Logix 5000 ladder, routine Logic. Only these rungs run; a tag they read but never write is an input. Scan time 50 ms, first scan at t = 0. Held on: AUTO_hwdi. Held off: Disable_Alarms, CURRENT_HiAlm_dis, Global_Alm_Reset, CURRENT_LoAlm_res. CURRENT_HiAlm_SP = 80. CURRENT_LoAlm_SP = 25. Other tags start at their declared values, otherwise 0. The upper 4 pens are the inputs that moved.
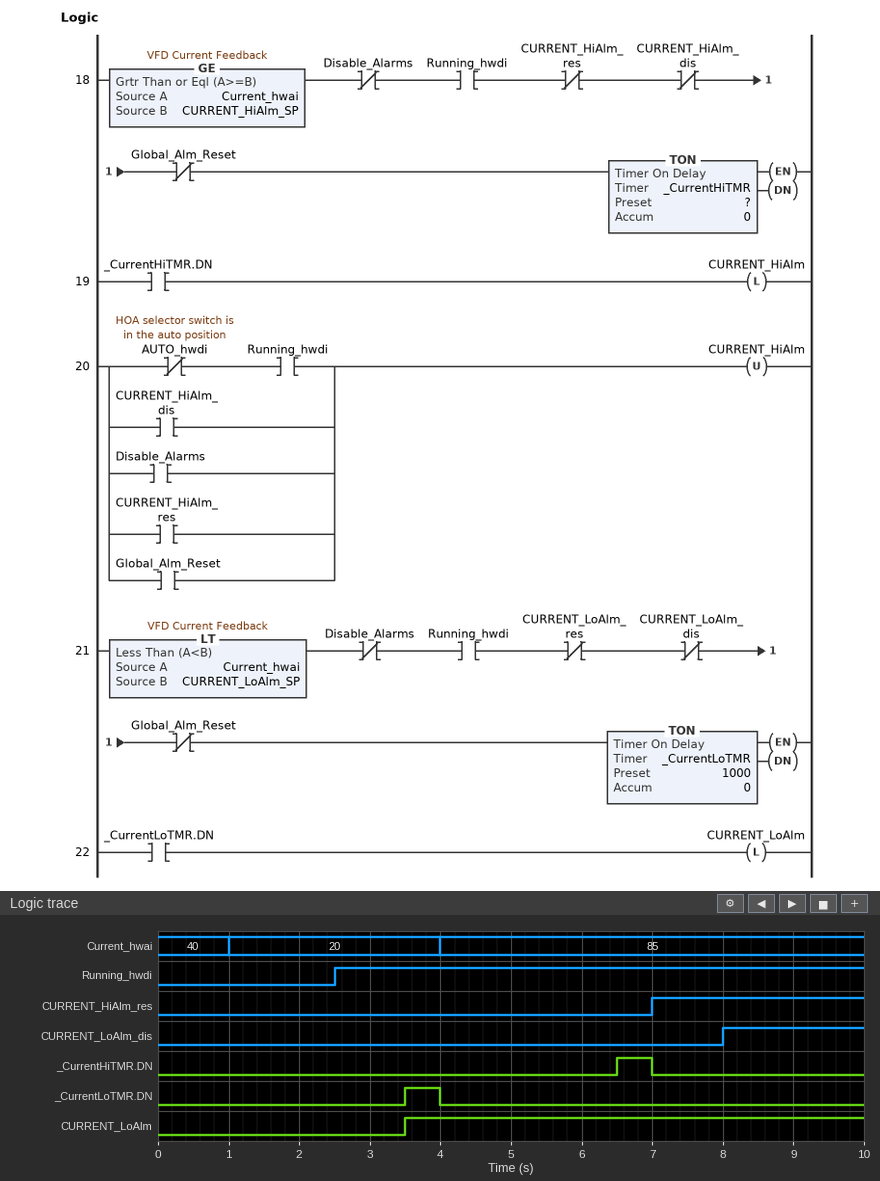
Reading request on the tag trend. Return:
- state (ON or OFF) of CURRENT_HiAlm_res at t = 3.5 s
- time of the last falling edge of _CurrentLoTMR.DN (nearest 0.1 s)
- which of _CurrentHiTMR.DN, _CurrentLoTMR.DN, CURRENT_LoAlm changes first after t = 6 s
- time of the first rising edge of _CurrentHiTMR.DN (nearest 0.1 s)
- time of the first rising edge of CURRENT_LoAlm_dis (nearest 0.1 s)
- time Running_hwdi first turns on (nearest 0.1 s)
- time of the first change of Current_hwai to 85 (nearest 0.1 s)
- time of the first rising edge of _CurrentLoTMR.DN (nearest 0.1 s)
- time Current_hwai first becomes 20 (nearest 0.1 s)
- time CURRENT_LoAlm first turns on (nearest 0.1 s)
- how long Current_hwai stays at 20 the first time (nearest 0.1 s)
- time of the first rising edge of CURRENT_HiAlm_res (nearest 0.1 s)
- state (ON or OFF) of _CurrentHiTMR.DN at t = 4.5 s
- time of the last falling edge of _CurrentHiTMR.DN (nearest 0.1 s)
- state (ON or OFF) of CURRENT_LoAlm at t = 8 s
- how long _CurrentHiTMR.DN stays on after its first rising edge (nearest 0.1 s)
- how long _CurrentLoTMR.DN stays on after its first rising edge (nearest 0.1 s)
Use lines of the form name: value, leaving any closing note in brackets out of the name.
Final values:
state (ON or OFF) of CURRENT_HiAlm_res at t = 3.5 s: OFF
time of the last falling edge of _CurrentLoTMR.DN: 4.0 s
which of _CurrentHiTMR.DN, _CurrentLoTMR.DN, CURRENT_LoAlm changes first after t = 6 s: _CurrentHiTMR.DN
time of the first rising edge of _CurrentHiTMR.DN: 6.5 s
time of the first rising edge of CURRENT_LoAlm_dis: 8.0 s
time Running_hwdi first turns on: 2.5 s
time of the first change of Current_hwai to 85: 4.0 s
time of the first rising edge of _CurrentLoTMR.DN: 3.5 s
time Current_hwai first becomes 20: 1.0 s
time CURRENT_LoAlm first turns on: 3.5 s
how long Current_hwai stays at 20 the first time: 3.0 s
time of the first rising edge of CURRENT_HiAlm_res: 7.0 s
state (ON or OFF) of _CurrentHiTMR.DN at t = 4.5 s: OFF
time of the last falling edge of _CurrentHiTMR.DN: 7.0 s
state (ON or OFF) of CURRENT_LoAlm at t = 8 s: ON
how long _CurrentHiTMR.DN stays on after its first rising edge: 0.5 s
how long _CurrentLoTMR.DN stays on after its first rising edge: 0.5 s
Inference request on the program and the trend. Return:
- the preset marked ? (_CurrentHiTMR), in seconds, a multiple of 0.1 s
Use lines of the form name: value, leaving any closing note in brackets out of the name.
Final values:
the preset marked ? (_CurrentHiTMR), in seconds, a multiple of 0.1 s: 2.5 s
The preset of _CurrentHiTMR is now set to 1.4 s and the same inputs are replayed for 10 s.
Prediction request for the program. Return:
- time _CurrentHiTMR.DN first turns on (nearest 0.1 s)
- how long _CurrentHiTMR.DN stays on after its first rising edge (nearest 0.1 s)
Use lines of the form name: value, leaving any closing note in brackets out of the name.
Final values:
time _CurrentHiTMR.DN first turns on: 5.4 s
how long _CurrentHiTMR.DN stays on after its first rising edge: 1.6 s
